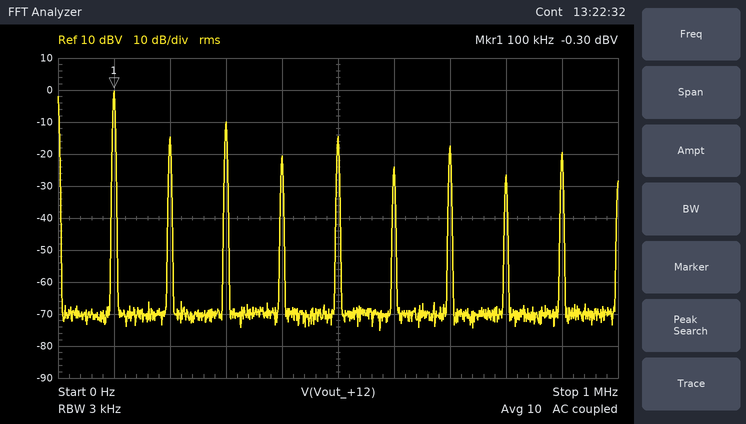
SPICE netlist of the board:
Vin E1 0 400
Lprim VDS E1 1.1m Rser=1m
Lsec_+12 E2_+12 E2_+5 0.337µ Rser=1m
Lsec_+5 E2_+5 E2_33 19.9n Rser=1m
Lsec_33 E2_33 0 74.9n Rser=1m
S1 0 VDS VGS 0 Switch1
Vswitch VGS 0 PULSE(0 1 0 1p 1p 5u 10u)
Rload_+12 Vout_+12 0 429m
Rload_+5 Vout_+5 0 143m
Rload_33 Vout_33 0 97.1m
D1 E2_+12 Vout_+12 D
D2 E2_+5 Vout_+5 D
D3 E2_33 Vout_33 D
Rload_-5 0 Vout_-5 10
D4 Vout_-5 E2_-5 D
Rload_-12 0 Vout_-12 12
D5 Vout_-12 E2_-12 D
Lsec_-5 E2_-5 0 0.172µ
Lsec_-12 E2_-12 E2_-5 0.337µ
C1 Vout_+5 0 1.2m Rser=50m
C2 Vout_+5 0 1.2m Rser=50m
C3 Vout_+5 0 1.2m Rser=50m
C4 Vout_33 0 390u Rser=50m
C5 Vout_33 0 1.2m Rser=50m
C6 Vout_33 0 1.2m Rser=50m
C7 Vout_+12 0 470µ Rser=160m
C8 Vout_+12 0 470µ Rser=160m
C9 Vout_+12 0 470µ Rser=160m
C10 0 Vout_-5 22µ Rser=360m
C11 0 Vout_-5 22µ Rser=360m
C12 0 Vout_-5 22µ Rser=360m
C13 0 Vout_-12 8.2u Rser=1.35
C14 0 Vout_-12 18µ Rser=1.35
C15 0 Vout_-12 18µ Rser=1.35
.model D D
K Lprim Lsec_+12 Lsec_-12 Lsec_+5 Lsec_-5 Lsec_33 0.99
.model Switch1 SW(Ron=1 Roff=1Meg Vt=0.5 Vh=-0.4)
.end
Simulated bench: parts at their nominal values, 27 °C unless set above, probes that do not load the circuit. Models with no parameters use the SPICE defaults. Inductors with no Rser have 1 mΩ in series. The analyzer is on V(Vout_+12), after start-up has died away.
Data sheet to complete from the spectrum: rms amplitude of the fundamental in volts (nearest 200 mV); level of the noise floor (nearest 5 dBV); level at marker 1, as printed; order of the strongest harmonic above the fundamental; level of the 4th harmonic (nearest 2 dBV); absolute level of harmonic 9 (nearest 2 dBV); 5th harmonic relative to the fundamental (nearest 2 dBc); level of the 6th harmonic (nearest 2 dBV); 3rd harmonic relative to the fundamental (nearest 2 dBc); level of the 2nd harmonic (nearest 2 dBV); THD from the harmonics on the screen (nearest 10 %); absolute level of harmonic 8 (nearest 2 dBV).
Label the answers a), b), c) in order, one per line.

a) 1.0 V
b) -70 dBV
c) -0.30 dBV
d) 3
e) -20 dBV
f) -20 dBV
g) -14 dBc
h) -24 dBV
i) -10 dBc
j) -14 dBV
k) 50 %
l) -26 dBV
